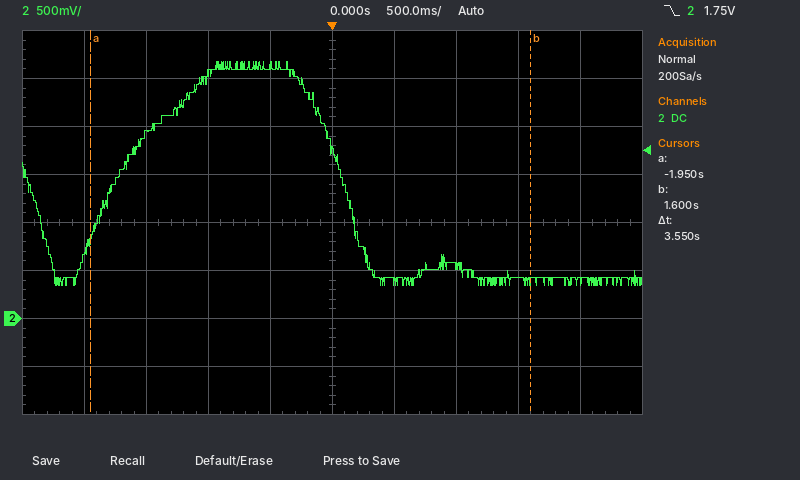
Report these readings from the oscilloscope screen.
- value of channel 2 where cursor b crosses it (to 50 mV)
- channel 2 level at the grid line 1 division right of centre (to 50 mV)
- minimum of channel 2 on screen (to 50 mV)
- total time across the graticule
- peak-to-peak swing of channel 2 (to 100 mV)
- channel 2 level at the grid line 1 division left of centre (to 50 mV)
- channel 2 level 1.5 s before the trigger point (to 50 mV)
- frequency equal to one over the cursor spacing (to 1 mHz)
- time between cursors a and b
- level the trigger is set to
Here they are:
400 mV
400 mV
350 mV
5 s
2.30 V
2.65 V
1.90 V
282 mHz
3.55 s
1.75 V
